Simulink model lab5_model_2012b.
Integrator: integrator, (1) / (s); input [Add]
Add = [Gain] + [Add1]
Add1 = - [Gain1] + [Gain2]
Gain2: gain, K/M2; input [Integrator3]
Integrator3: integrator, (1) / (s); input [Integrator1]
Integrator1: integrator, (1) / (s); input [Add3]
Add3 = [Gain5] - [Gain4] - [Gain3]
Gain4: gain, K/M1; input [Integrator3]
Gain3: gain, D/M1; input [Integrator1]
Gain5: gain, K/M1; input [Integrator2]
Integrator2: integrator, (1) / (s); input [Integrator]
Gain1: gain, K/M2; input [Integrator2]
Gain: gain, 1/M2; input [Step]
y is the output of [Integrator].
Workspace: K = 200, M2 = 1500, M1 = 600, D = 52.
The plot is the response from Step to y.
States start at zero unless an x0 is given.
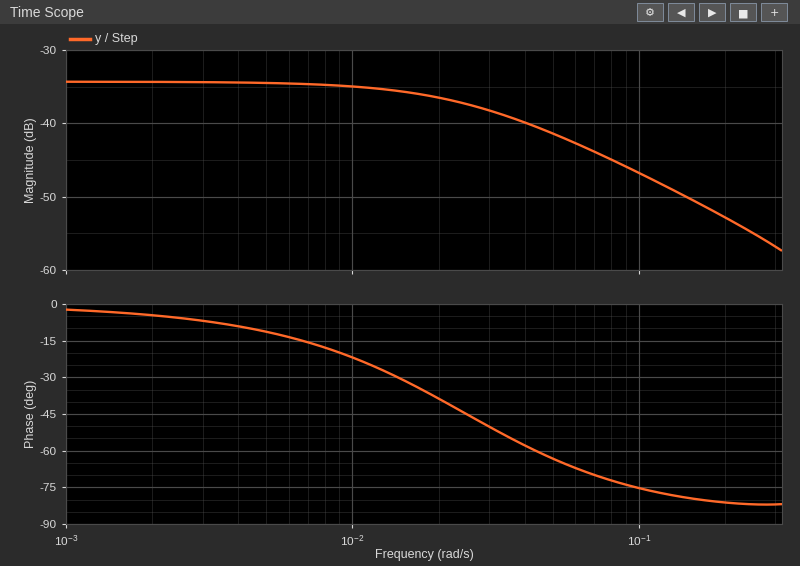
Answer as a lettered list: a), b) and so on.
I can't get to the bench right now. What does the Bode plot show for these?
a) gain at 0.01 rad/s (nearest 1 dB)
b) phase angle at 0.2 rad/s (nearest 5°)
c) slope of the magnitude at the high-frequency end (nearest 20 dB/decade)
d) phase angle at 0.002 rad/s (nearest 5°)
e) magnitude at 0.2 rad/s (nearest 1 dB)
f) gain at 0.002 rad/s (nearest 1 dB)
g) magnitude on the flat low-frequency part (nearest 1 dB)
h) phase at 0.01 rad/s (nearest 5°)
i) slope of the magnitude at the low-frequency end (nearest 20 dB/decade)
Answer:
a) -35 dB
b) -80°
c) -20 dB/decade
d) -5°
e) -53 dB
f) -34 dB
g) -34 dB
h) -20°
i) 0 dB/decade
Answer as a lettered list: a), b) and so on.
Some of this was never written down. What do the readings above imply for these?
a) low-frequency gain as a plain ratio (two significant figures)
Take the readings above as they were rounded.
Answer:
a) 0.020
